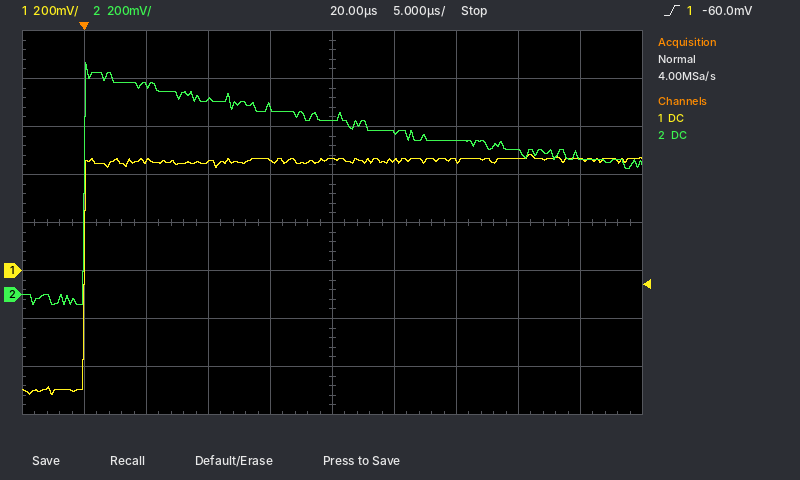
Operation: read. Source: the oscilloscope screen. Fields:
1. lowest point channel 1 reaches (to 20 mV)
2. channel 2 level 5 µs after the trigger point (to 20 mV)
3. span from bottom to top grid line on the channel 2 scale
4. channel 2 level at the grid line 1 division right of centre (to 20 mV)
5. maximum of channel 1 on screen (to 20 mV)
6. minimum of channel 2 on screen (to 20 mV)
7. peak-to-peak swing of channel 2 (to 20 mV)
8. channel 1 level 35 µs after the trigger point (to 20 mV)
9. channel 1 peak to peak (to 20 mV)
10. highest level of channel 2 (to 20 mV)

-520 mV
880 mV
1.6 V
680 mV
480 mV
-40 mV
1.00 V
460 mV
1.00 V
960 mV
